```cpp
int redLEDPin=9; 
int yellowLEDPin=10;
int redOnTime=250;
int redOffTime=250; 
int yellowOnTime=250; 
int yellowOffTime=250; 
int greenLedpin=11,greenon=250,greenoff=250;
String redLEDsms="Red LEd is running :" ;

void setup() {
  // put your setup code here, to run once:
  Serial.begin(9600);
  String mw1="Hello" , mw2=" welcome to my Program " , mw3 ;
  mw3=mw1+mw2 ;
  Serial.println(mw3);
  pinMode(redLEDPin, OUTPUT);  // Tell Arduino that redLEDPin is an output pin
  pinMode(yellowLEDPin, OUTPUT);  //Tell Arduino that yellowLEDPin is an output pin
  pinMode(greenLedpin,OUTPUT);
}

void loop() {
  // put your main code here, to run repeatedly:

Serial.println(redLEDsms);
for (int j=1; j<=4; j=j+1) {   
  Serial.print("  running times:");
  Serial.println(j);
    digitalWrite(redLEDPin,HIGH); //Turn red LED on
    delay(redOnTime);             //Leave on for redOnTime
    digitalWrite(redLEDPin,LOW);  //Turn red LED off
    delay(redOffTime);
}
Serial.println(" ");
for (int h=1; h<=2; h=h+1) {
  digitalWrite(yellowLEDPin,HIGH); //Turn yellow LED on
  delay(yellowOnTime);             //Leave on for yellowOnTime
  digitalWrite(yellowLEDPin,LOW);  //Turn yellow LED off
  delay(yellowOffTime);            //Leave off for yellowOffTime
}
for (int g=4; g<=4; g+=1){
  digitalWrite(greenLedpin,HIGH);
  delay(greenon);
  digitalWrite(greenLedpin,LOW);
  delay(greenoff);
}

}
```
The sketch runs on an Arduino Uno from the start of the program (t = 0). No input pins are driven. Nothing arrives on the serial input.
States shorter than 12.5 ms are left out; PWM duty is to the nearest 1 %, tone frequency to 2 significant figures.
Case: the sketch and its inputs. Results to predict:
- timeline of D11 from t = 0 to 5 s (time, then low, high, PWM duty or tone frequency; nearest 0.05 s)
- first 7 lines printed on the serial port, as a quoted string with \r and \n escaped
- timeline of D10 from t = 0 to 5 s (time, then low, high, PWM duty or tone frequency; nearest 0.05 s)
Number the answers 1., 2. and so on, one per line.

1. 0 s low; 3 s high; 3.25 s low
2. "Hello welcome to my Program \r\nRed LEd is running :\r\n  running times:1\r\n  running times:2\r\n  running times:3\r\n  running times:4\r\n \r\n"
3. 0 s low; 2 s high; 2.25 s low; 2.5 s high; 2.75 s low
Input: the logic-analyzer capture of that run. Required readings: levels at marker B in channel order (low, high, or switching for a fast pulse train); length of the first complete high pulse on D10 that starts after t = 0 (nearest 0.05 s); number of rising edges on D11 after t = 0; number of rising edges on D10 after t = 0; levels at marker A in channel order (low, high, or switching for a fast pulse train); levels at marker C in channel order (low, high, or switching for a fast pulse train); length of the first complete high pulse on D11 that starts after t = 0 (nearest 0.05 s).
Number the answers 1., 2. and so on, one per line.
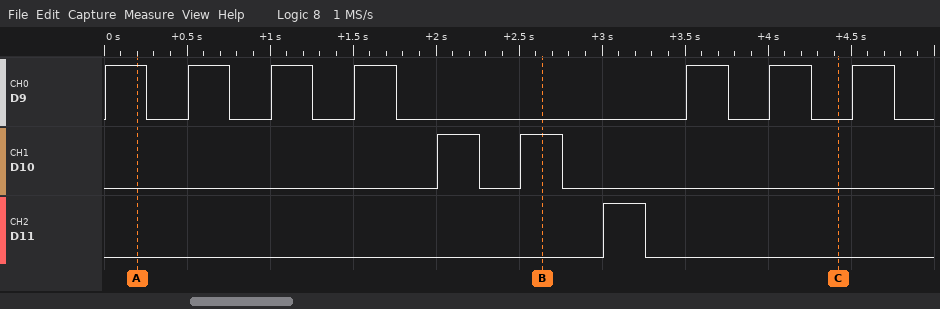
1. D9 low, D10 high, D11 low
2. 0.25 s
3. 1
4. 2
5. D9 high, D10 low, D11 low
6. D9 low, D10 low, D11 low
7. 0.25 s
